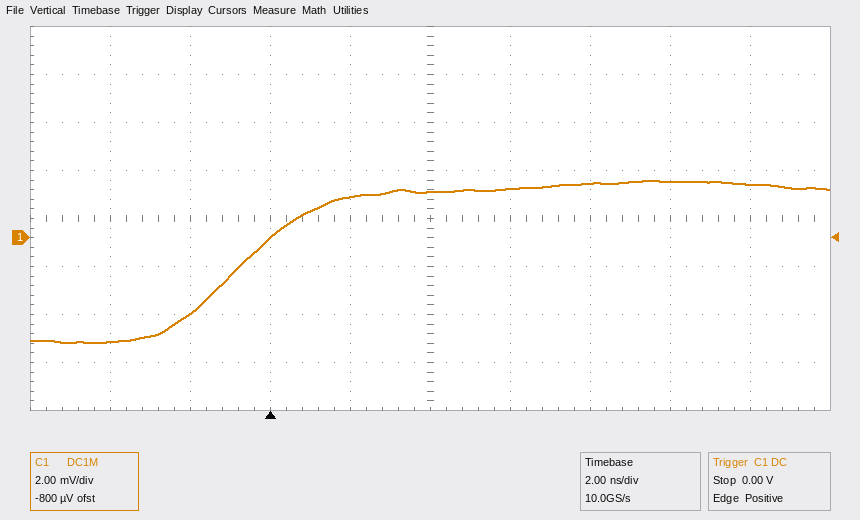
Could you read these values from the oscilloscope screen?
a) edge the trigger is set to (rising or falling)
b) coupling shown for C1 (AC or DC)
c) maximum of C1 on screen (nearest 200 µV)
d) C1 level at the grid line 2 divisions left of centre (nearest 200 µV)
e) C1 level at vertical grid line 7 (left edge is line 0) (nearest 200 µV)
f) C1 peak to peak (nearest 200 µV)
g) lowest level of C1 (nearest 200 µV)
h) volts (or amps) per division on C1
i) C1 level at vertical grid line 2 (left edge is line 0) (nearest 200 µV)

rising
DC
2.4 mV
0.0 mV
2.2 mV
6.8 mV
-4.4 mV
2 mV
-3.2 mV
